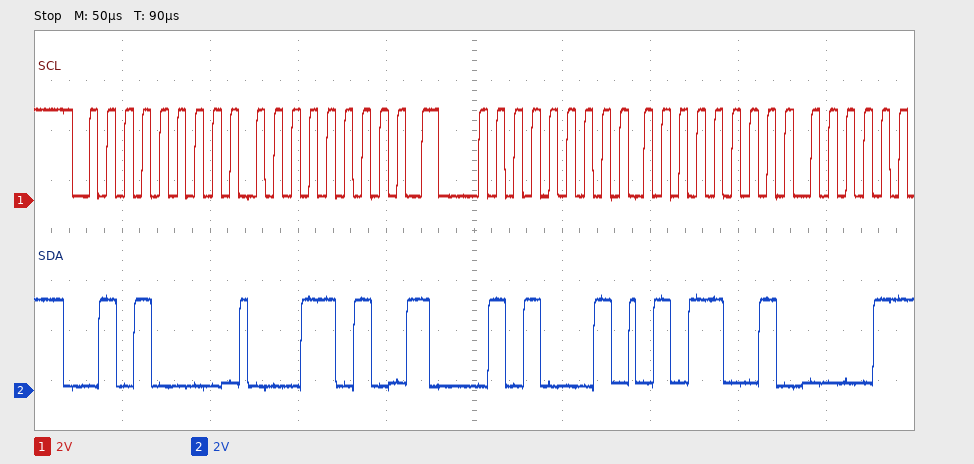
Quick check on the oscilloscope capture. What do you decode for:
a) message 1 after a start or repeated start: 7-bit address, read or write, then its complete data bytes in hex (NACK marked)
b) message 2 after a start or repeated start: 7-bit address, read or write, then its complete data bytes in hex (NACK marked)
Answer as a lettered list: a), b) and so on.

a) 0x28 write: 1A
b) 0x28 read: 59
